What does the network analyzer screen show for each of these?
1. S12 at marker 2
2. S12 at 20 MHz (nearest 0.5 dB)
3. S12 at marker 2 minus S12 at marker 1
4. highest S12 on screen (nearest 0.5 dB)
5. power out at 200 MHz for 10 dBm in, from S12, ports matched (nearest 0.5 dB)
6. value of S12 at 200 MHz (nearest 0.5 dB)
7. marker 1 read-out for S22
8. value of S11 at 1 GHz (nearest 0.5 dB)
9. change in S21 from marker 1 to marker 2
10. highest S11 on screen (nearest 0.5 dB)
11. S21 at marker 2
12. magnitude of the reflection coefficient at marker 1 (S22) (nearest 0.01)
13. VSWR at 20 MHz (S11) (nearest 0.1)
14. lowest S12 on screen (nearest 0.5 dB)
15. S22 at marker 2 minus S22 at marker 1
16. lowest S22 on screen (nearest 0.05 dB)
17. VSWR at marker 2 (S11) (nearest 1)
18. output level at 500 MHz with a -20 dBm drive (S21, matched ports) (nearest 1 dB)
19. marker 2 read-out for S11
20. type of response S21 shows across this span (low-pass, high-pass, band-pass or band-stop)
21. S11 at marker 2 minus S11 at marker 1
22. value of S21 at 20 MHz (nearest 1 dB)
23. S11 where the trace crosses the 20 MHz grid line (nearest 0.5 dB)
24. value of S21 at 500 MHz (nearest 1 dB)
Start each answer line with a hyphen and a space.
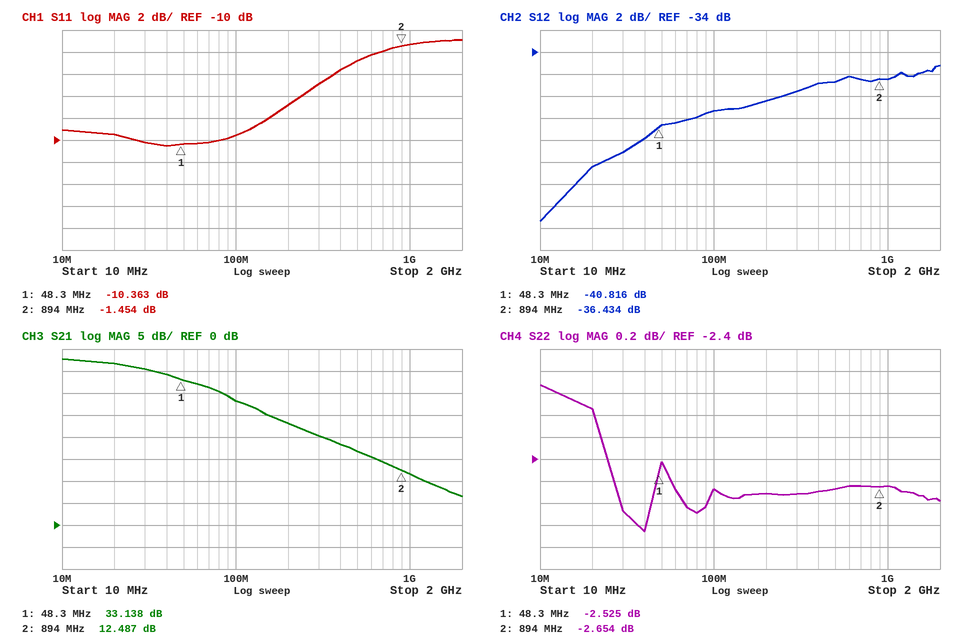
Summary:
- -36.434 dB
- -44.5 dB
- 4.382 dB
- -35.0 dB
- -28.5 dBm
- -38.5 dB
- -2.525 dB
- -1.5 dB
- -20.651 dB
- -1.0 dB
- 12.487 dB
- 0.75
- 2.0
- -49.5 dB
- -0.129 dB
- -3.05 dB
- 12
- -3 dBm
- -1.454 dB
- low-pass
- 8.909 dB
- 37 dB
- -9.5 dB
- 17 dB
